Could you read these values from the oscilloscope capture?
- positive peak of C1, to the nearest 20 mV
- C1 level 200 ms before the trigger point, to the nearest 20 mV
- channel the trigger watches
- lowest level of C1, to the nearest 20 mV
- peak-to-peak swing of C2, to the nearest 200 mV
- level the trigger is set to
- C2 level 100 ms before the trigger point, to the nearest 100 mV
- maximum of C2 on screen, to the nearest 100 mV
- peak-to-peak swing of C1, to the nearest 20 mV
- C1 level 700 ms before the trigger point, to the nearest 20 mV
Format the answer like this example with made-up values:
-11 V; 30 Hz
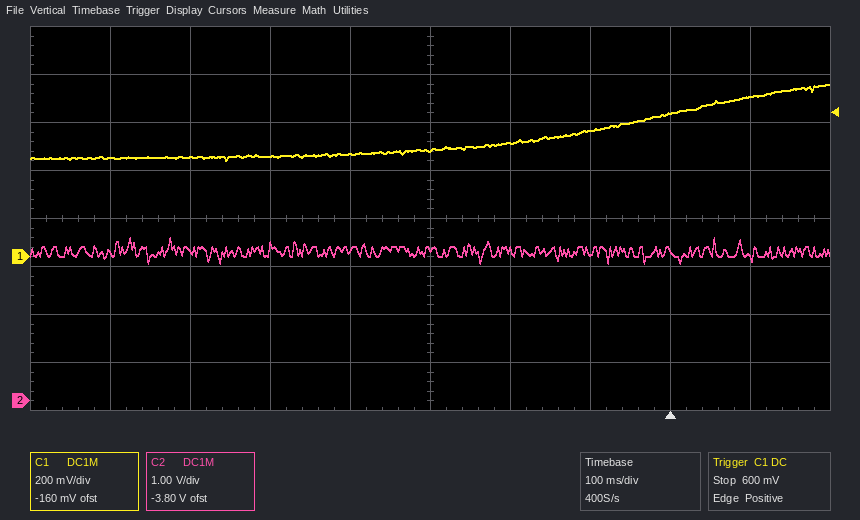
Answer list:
720 mV; 480 mV; C1; 400 mV; 600 mV; 600 mV; 3.1 V; 3.4 V; 320 mV; 420 mV
